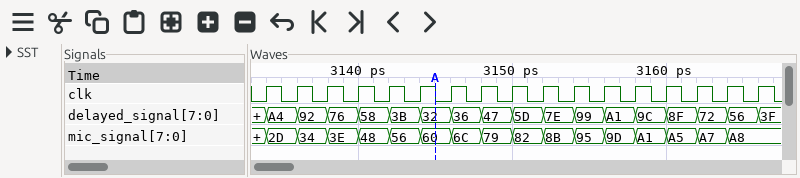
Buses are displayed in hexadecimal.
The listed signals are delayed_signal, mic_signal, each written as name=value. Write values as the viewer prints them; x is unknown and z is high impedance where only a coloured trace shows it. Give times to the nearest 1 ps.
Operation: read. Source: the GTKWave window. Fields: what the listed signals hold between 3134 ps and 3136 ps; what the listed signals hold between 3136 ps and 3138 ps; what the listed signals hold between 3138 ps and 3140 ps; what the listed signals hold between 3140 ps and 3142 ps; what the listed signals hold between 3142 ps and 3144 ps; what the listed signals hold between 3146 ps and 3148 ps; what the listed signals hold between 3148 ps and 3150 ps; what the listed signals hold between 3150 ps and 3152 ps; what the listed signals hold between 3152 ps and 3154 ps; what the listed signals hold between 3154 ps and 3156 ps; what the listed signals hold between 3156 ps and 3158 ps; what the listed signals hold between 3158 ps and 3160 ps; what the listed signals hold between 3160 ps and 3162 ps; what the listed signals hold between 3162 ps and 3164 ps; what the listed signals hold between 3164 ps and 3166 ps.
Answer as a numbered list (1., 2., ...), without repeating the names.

1. delayed_signal=A4, mic_signal=2D
2. delayed_signal=92, mic_signal=34
3. delayed_signal=76, mic_signal=3E
4. delayed_signal=58, mic_signal=48
5. delayed_signal=3B, mic_signal=56
6. delayed_signal=36, mic_signal=6C
7. delayed_signal=47, mic_signal=79
8. delayed_signal=5D, mic_signal=82
9. delayed_signal=7E, mic_signal=8B
10. delayed_signal=99, mic_signal=95
11. delayed_signal=A1, mic_signal=9D
12. delayed_signal=9C, mic_signal=A1
13. delayed_signal=8F, mic_signal=A5
14. delayed_signal=72, mic_signal=A7
15. delayed_signal=56, mic_signal=A8
